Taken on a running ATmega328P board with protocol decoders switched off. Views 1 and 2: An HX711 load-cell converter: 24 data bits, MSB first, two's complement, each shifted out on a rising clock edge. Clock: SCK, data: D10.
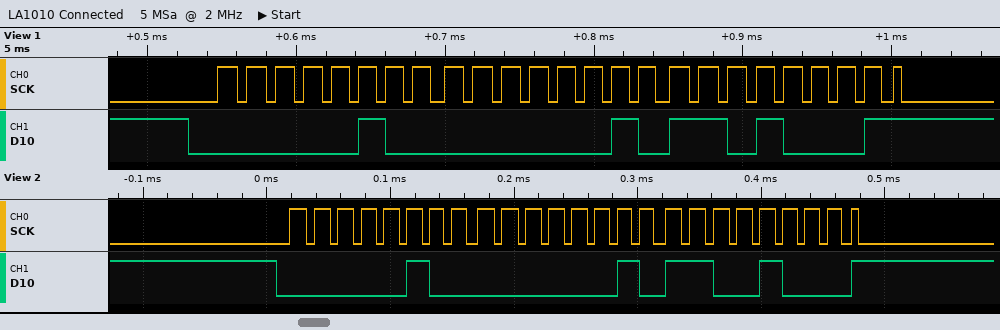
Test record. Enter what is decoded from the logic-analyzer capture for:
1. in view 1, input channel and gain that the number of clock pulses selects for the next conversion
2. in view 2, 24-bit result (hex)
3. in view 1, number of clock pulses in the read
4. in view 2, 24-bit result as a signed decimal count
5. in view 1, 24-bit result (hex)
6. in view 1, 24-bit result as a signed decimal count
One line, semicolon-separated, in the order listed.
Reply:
channel A, gain 128; 0x0402C8; 25; 262856; 0x0402D1; 262865
